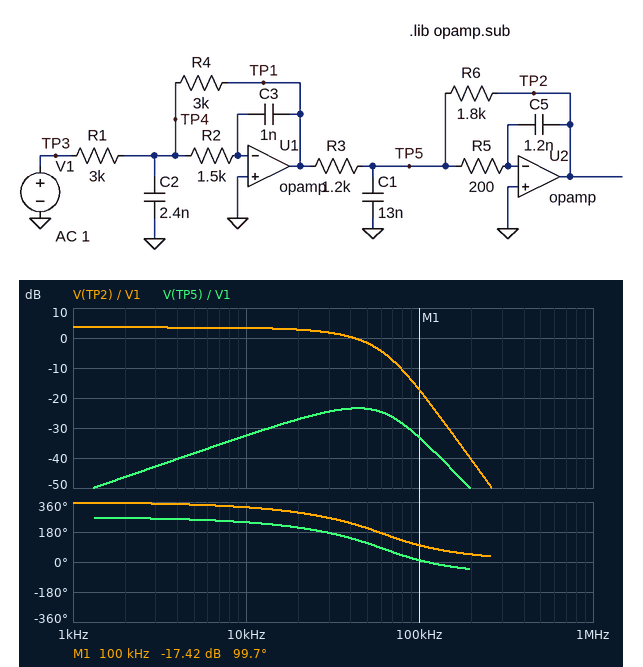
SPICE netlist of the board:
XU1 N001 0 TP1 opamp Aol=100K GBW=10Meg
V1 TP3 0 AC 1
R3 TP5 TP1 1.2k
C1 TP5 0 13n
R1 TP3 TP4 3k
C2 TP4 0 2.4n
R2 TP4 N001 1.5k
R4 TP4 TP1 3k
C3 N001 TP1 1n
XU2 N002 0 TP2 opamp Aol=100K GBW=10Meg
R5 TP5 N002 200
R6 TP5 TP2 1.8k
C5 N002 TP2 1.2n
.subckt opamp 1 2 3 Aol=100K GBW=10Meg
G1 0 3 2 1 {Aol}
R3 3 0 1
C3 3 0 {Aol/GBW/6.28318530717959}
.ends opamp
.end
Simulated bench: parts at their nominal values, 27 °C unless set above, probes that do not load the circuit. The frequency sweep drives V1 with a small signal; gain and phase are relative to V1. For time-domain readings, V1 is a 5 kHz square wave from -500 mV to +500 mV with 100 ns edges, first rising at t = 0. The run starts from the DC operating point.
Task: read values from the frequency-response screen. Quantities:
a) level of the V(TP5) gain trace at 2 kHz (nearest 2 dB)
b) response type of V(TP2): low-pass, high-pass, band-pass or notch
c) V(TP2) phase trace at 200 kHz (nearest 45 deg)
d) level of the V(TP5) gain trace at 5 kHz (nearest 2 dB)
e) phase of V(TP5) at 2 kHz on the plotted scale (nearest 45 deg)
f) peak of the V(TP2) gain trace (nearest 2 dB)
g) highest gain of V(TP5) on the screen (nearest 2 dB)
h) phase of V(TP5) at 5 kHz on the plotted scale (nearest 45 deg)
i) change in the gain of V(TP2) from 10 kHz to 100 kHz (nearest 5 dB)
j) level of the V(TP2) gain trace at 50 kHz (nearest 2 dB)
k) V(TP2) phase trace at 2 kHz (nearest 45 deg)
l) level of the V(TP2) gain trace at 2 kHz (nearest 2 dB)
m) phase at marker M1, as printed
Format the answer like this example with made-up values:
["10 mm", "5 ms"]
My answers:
["-46 dB", "low-pass", "45 deg", "-38 dB", "270 deg", "4 dB", "-24 dB", "270 deg", "-20 dB", "-2 dB", "360 deg", "4 dB", "99.7 deg"]
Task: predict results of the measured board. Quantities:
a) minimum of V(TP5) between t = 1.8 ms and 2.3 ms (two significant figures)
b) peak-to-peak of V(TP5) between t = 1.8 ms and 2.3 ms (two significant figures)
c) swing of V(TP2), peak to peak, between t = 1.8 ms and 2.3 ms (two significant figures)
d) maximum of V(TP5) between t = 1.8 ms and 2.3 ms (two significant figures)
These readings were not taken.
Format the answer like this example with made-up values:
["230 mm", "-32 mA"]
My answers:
["-42 mV", "84 mV", "1.5 V", "42 mV"]
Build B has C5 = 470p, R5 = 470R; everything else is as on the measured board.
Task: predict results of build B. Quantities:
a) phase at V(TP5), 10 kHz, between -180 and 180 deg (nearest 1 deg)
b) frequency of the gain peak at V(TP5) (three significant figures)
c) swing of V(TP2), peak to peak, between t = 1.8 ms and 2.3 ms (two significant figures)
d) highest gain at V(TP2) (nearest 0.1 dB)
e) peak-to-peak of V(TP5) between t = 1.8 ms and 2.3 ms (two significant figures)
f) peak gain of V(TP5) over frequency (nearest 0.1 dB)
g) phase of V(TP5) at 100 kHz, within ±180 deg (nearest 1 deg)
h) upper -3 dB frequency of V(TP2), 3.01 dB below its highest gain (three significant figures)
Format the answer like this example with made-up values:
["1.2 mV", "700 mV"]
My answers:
["-117 deg", "59.1 kHz", "1.7 V", "3.5 dB", "100 mV", "-20.0 dB", "-5 deg", "62.3 kHz"]
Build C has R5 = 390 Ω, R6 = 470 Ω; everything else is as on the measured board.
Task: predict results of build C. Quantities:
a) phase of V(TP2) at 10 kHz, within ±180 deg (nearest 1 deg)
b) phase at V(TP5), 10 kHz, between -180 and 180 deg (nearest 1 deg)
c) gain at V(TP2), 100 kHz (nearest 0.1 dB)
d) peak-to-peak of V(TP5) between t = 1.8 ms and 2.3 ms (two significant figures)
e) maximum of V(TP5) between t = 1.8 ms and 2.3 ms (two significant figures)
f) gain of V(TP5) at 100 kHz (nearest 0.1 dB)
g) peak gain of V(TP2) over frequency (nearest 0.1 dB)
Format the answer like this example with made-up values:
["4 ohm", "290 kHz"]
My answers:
["-26 deg", "-116 deg", "-20.1 dB", "54 mV", "27 mV", "-30.4 dB", "-8.1 dB"]
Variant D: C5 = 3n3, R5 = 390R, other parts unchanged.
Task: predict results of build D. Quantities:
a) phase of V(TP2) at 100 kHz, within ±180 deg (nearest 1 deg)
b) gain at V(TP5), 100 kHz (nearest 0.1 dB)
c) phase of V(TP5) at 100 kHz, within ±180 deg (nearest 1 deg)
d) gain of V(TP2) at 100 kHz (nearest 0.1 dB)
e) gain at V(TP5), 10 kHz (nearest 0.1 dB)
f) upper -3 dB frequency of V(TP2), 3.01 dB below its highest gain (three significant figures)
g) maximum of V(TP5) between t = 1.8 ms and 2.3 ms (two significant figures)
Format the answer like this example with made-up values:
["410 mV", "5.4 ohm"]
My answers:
["75 deg", "-34.1 dB", "-14 deg", "-32.4 dB", "-18.9 dB", "19.9 kHz", "120 mV"]
